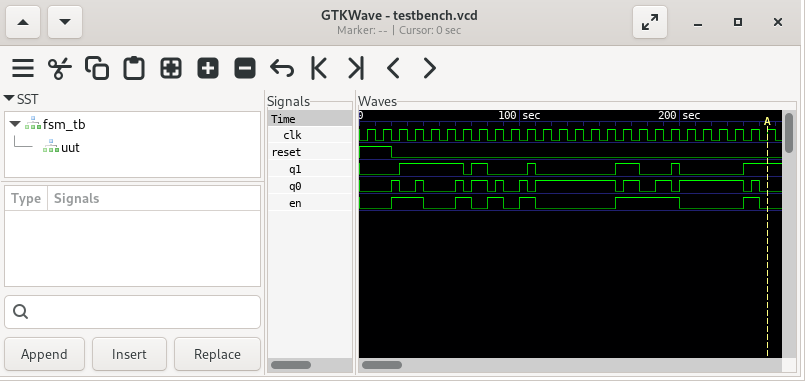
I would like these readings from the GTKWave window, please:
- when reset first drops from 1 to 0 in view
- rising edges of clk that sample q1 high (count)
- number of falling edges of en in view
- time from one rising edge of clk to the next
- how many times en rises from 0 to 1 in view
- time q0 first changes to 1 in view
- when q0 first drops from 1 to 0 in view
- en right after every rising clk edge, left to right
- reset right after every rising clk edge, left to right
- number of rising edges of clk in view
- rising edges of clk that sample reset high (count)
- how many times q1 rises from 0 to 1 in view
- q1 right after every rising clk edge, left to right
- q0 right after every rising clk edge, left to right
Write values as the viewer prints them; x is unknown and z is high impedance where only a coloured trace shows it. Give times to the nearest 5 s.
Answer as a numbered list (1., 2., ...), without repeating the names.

1. 20 s
2. 9
3. 6
4. 10 s
5. 6
6. 20 s
7. 25 s
8. 0 0 1 1 0 0 1 0 1 0 1 0 0 0 0 0 1 1 1 1 0 0 0 0 1 0
9. 1 1 0 0 0 0 0 0 0 0 0 0 0 0 0 0 0 0 0 0 0 0 0 0 0 0
10. 26
11. 2
12. 6
13. 0 0 1 1 1 1 0 1 0 0 1 0 0 0 0 0 1 0 0 1 0 0 0 0 1 1
14. 0 0 0 1 0 0 0 1 1 0 0 1 1 1 1 1 1 0 1 0 1 1 1 1 1 0
